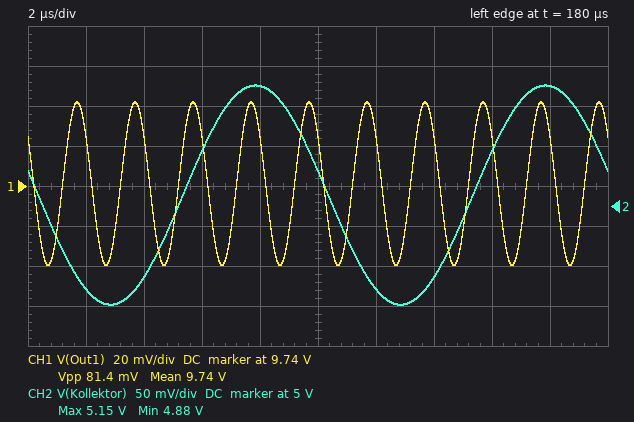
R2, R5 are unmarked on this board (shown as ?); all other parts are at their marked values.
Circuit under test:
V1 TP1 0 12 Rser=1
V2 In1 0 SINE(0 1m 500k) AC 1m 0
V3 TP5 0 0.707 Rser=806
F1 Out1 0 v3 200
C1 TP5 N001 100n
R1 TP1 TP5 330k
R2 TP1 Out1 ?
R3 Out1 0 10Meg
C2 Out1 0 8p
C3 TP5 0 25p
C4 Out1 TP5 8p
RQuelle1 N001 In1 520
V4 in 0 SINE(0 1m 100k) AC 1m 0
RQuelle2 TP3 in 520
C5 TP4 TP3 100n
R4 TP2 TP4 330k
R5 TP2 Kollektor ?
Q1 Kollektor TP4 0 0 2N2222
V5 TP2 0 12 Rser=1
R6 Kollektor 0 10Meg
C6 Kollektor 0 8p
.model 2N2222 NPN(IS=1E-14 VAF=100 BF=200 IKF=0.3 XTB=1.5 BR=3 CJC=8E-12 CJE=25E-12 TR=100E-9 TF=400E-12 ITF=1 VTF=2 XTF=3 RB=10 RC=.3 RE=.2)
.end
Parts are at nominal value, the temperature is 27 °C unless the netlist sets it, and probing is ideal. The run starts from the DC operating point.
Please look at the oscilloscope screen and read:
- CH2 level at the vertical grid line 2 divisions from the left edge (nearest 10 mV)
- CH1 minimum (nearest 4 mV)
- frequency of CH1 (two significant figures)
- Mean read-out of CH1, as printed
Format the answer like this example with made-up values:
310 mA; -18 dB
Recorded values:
4.91 V; 9.700 V; 500 kHz; 9.74 V
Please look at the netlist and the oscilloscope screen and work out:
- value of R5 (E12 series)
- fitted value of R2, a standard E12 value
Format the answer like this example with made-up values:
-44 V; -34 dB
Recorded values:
1 kΩ; 330 Ω
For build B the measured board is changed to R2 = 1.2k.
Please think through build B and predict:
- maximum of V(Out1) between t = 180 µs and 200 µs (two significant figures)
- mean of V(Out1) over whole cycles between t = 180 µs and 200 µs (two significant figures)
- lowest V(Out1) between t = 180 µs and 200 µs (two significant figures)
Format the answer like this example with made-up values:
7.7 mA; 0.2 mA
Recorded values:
3.9 V; 3.8 V; 3.7 V
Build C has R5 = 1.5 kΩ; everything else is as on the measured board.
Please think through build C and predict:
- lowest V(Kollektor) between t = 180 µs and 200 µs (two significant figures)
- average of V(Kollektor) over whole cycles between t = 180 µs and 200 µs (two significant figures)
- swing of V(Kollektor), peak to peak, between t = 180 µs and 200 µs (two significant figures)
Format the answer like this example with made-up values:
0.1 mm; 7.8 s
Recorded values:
1.7 V; 1.8 V; 360 mV
